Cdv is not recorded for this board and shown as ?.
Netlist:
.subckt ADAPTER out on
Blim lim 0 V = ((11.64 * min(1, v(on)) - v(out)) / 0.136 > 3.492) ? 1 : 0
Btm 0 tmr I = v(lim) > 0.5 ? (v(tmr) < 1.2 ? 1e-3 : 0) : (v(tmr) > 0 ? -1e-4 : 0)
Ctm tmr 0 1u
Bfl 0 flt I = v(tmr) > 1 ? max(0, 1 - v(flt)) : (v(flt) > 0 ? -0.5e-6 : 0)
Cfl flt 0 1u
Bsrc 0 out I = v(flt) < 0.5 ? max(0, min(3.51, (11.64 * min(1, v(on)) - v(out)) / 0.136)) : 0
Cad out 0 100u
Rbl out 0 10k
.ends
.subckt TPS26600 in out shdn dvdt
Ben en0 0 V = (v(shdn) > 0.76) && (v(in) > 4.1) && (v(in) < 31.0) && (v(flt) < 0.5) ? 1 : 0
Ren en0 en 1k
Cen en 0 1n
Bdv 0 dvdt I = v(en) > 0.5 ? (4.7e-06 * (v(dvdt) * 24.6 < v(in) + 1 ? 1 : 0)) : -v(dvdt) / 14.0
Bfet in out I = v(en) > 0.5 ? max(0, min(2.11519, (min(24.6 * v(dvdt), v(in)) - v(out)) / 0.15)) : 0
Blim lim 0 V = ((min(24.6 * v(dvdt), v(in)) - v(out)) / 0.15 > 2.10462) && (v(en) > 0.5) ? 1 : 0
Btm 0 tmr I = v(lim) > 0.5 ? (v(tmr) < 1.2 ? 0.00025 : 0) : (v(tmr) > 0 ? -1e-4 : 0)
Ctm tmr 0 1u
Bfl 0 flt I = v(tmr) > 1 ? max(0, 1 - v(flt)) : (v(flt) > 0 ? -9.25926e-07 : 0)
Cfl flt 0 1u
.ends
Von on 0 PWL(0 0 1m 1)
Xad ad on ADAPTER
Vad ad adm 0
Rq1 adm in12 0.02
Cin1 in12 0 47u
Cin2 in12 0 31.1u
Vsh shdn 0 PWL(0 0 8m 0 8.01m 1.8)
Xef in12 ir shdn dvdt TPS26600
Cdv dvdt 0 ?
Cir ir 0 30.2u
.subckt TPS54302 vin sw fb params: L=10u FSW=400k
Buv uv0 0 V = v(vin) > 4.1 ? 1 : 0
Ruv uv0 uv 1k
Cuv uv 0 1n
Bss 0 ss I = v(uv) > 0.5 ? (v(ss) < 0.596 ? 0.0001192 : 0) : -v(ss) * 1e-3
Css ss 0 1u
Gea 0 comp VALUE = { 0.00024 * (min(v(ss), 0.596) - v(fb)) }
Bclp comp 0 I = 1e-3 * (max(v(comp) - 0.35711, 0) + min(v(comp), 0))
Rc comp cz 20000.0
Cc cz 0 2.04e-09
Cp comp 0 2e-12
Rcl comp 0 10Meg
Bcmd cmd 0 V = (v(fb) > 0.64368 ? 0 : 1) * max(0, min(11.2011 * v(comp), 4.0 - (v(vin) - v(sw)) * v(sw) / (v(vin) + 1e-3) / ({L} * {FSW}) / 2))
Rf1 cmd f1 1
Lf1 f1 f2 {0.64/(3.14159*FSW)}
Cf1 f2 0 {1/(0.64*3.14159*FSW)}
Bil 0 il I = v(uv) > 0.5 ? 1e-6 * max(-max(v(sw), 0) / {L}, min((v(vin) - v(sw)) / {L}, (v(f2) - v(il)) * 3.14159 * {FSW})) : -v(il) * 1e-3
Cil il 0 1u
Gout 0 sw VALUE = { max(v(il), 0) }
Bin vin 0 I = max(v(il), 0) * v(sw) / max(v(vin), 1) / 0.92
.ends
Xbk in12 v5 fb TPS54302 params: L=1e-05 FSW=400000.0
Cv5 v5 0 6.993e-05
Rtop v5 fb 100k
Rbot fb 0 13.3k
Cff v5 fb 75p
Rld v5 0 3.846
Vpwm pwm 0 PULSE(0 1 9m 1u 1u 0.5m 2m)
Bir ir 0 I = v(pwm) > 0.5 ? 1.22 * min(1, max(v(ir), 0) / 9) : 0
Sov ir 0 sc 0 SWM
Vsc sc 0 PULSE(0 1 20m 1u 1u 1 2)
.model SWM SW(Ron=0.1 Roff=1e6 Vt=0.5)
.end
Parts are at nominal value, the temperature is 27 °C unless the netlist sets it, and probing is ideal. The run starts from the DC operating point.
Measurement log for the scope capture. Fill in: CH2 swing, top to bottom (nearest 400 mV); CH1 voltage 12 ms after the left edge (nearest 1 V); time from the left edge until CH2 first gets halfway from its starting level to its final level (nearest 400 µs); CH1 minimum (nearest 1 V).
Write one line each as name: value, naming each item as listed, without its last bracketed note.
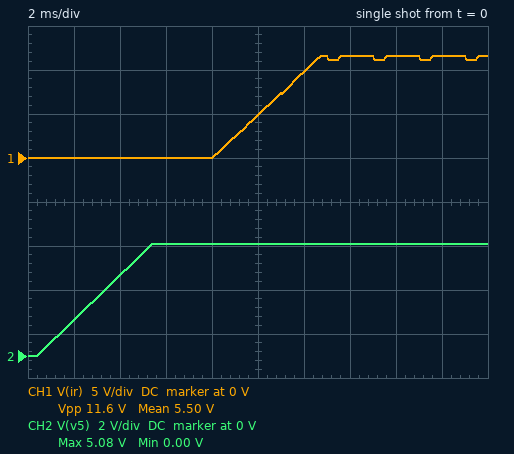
CH2 swing, top to bottom: 5.2 V
CH1 voltage 12 ms after the left edge: 10 V
time from the left edge until CH2 first gets halfway from its starting level to its final level: 2.8 ms
CH1 minimum: 0 V
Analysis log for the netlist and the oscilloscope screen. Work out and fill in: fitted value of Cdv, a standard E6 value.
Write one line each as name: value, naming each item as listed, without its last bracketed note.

fitted value of Cdv, a standard E6 value: 47 nF
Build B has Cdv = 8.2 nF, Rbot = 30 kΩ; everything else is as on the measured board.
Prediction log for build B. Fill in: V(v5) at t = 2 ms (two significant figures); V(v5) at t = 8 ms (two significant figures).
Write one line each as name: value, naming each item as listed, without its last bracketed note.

V(v5) at t = 2 ms: 830 mV
V(v5) at t = 8 ms: 2.6 V
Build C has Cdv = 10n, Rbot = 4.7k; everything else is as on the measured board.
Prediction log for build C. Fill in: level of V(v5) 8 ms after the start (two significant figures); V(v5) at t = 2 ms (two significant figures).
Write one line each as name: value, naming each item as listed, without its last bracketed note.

level of V(v5) 8 ms after the start: 11 V
V(v5) at t = 2 ms: 4.3 V
